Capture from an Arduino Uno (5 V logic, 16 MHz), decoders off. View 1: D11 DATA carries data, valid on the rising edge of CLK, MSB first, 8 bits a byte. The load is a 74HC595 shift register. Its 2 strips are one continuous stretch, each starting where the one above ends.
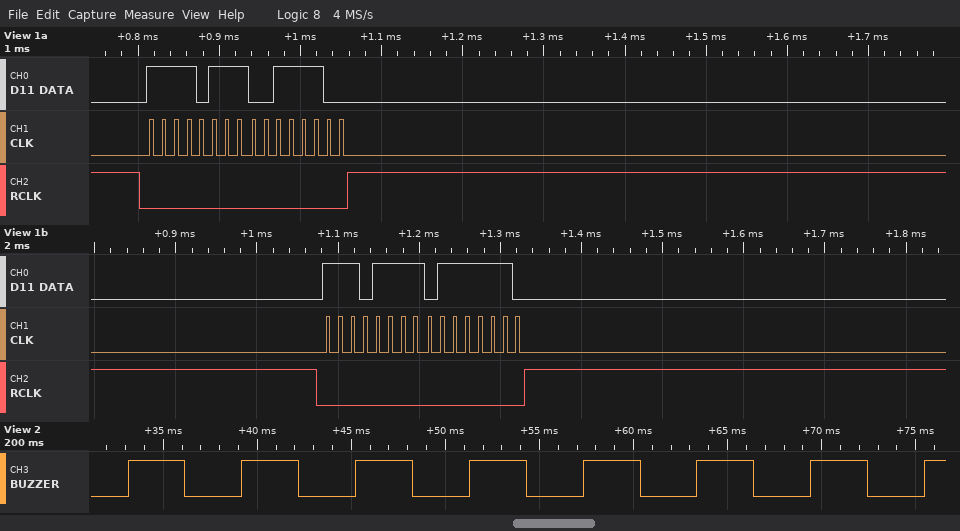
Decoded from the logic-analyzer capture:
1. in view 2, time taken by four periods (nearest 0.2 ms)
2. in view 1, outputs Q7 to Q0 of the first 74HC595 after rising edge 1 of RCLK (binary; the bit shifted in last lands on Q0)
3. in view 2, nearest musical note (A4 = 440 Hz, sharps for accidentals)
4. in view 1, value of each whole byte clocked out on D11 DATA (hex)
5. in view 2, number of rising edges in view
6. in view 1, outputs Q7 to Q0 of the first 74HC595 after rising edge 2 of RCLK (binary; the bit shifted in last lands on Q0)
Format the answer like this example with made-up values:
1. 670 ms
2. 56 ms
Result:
1. 24.2 ms
2. 00111100
3. E3
4. F7 3C EF 7E
5. 8
6. 01111110
